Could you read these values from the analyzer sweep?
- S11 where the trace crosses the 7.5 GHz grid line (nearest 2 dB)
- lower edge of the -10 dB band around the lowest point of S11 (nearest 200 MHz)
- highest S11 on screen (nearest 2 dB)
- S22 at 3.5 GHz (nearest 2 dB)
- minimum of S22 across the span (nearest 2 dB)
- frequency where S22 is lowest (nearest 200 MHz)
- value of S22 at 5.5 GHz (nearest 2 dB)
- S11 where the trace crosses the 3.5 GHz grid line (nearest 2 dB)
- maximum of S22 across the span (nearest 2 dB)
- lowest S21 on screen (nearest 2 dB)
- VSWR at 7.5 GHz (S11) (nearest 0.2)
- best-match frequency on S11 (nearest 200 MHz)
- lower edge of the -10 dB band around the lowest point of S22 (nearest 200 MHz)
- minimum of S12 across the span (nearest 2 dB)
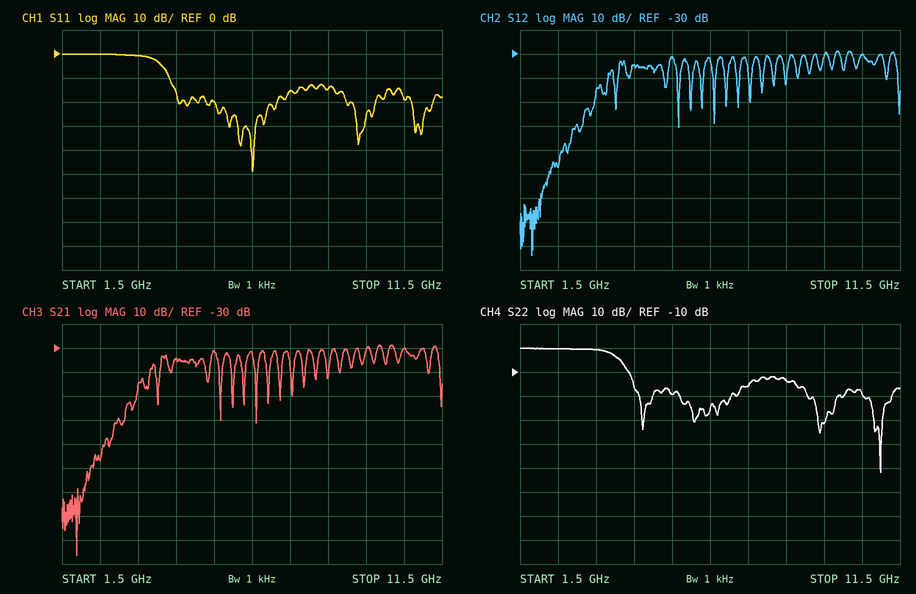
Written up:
-16 dB
4.4 GHz
0 dB
0 dB
-52 dB
11.0 GHz
-20 dB
0 dB
0 dB
-116 dB
1.4
6.6 GHz
4.4 GHz
-114 dB
